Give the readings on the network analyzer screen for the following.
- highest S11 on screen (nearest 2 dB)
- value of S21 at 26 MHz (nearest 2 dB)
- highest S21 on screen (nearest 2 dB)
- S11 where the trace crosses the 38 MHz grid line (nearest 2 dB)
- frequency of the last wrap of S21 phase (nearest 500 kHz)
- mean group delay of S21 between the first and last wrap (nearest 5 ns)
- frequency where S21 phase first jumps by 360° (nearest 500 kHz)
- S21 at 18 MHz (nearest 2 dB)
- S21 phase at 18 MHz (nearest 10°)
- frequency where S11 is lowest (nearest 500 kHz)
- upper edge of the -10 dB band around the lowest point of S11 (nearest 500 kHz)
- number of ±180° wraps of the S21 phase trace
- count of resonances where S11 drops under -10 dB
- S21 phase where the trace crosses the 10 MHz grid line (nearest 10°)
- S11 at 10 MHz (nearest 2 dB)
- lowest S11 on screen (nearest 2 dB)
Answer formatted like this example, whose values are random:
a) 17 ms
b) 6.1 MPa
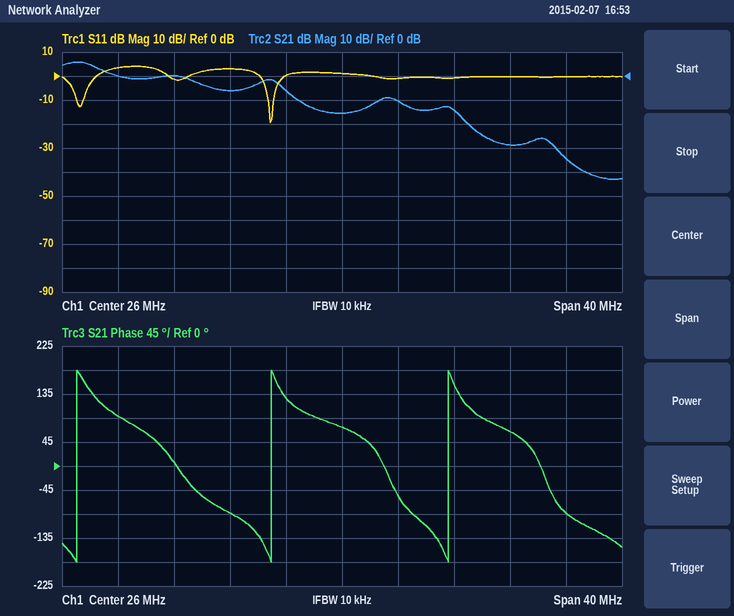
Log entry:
a) 4 dB
b) -16 dB
c) 6 dB
d) 0 dB
e) 33.5 MHz
f) 75 ns
g) 7.0 MHz
h) -6 dB
i) -90°
j) 21.0 MHz
k) 21.0 MHz
l) 3
m) 2
n) 90°
o) 4 dB
p) -20 dB
